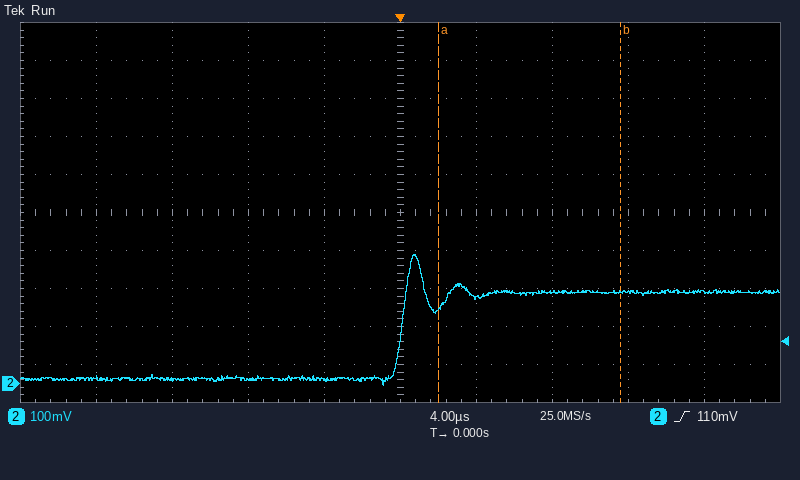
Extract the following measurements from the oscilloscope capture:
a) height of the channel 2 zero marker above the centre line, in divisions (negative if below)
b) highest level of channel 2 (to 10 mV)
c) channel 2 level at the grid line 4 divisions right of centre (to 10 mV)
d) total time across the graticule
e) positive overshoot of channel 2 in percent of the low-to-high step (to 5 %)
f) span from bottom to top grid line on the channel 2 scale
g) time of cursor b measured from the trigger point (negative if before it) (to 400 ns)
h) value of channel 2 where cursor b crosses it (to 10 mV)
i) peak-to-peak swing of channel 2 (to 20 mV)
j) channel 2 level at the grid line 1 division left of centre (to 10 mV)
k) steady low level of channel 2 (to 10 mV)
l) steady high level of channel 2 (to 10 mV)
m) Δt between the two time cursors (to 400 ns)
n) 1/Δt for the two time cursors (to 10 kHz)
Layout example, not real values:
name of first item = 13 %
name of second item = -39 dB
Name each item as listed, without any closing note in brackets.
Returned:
height of the channel 2 zero marker above the centre line, in divisions = -4.5 div
highest level of channel 2 = 340 mV
channel 2 level at the grid line 4 divisions right of centre = 240 mV
total time across the graticule = 40 µs
positive overshoot of channel 2 in percent of the low-to-high step = 45 %
span from bottom to top grid line on the channel 2 scale = 1 V
time of cursor b measured from the trigger point (negative if before it) = +11.6 µs
value of channel 2 where cursor b crosses it = 240 mV
peak-to-peak swing of channel 2 = 340 mV
channel 2 level at the grid line 1 division left of centre = 10 mV
steady low level of channel 2 = 10 mV
steady high level of channel 2 = 240 mV
Δt between the two time cursors = 9.6 µs
1/Δt for the two time cursors = 100 kHz
